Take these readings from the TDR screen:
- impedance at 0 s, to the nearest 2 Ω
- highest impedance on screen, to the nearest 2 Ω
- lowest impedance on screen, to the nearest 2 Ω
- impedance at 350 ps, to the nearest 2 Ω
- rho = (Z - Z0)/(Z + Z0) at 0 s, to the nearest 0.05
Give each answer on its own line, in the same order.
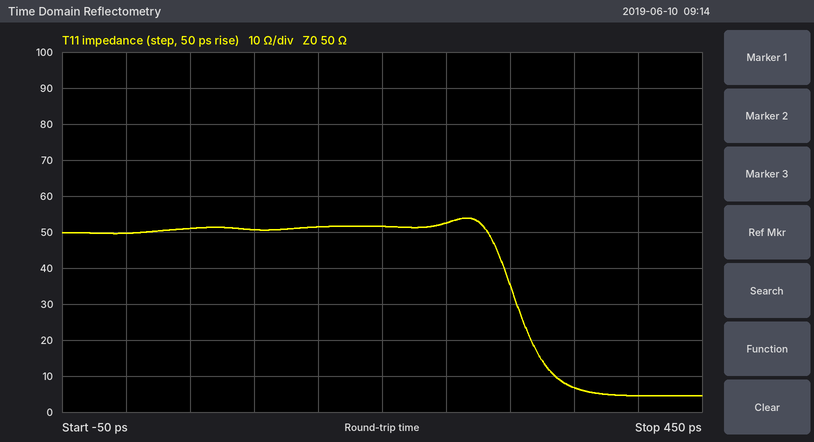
50 Ω
54 Ω
4 Ω
6 Ω
0.00
